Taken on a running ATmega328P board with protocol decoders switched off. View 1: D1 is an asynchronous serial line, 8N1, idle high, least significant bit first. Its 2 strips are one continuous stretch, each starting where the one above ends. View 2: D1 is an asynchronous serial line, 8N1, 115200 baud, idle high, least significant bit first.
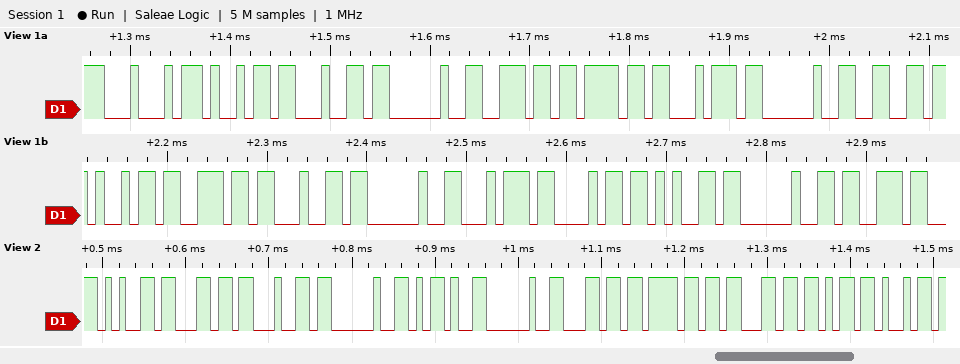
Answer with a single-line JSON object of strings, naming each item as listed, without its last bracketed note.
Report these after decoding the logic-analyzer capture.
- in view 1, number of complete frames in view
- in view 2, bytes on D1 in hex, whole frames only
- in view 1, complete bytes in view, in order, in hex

{"in view 1, number of complete frames in view": "18", "in view 2, bytes on D1 in hex, whole frames only": "0x65 0x6C 0x64 0x20 0x2D 0x20 0x6C 0x6F 0x63 0x6B 0x69", "in view 1, complete bytes in view, in order, in hex": "44 69 64 20 6E 6F 74 20 66 69 6E 64 20 74 68 65 20 73"}
